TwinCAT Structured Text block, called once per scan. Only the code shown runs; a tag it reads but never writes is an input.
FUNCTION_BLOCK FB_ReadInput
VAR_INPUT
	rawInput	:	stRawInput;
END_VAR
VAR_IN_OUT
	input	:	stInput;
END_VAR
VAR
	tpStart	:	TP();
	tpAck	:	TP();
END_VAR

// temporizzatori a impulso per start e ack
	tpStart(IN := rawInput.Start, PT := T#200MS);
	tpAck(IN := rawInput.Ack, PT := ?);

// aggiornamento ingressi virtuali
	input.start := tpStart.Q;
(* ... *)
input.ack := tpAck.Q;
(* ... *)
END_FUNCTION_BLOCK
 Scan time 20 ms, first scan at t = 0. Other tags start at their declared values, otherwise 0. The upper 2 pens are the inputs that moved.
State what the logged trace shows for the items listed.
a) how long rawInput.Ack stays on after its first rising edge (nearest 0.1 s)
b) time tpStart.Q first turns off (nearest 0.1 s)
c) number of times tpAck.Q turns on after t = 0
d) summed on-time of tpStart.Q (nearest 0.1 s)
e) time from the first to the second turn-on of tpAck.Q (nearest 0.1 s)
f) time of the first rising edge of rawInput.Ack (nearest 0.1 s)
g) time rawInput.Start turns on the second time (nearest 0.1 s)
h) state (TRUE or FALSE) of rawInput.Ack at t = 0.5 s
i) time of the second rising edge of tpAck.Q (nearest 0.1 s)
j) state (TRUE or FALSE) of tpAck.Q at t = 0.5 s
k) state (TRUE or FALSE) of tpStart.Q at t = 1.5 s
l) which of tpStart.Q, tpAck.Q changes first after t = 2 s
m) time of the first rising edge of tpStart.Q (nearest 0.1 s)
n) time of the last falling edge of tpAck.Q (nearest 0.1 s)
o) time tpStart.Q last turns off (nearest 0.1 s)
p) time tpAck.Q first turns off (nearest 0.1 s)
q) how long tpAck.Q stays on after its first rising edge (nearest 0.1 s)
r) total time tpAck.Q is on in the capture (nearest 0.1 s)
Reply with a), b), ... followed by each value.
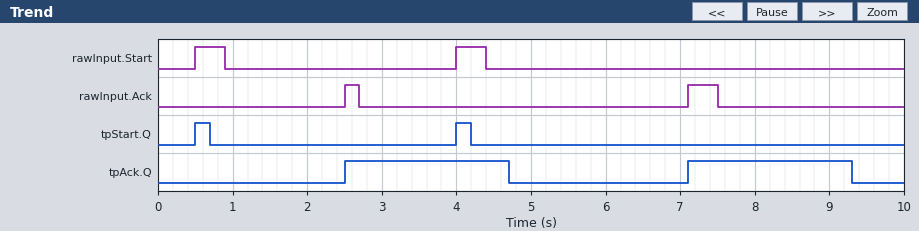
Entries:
a) 0.2 s
b) 0.7 s
c) 2
d) 0.4 s
e) 4.6 s
f) 2.5 s
g) 4.0 s
h) FALSE
i) 7.1 s
j) FALSE
k) FALSE
l) tpAck.Q
m) 0.5 s
n) 9.3 s
o) 4.2 s
p) 4.7 s
q) 2.2 s
r) 4.4 s
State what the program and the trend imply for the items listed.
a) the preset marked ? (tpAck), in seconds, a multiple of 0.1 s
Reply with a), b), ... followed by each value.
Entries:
a) 2.2 s
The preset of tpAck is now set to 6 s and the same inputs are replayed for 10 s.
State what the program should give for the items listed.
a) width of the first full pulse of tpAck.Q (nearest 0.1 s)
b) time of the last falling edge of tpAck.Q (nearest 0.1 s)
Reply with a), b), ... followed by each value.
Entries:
a) 6.0 s
b) 8.5 s
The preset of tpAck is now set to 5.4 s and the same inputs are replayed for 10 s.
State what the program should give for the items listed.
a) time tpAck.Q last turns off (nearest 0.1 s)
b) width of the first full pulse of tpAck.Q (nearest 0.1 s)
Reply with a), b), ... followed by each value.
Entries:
a) 7.9 s
b) 5.4 s
